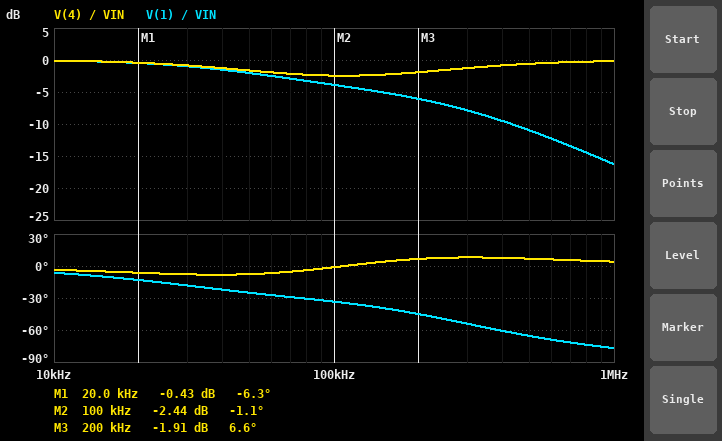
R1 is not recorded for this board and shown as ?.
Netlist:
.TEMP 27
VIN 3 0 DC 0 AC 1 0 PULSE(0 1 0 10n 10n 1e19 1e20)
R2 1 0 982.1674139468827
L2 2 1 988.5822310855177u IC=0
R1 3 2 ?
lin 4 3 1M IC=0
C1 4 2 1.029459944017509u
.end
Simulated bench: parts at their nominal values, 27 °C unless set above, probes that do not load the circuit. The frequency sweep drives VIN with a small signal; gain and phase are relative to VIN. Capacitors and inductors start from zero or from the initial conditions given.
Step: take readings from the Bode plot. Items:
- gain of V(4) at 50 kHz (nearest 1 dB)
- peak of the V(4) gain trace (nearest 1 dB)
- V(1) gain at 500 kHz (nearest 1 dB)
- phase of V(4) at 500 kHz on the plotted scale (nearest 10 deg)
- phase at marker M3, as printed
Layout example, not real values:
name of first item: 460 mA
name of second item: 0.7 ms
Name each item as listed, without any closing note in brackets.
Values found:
gain of V(4) at 50 kHz: -2 dB
peak of the V(4) gain trace: 0 dB
V(1) gain at 500 kHz: -11 dB
phase of V(4) at 500 kHz on the plotted scale: 10 deg
phase at marker M3, as printed: 6.6 deg
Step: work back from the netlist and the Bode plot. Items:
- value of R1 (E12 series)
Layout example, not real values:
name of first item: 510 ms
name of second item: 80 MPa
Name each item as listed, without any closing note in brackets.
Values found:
value of R1: 470 Ω
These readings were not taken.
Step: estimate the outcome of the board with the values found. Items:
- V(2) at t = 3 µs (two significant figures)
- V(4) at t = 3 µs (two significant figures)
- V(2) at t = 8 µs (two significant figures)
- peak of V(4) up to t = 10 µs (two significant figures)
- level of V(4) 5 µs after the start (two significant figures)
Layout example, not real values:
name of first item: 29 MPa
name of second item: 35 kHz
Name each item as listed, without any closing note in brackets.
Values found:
V(2) at t = 3 µs: 850 mV
V(4) at t = 3 µs: 850 mV
V(2) at t = 8 µs: 960 mV
peak of V(4) up to t = 10 µs: 1.0 V
level of V(4) 5 µs after the start: 920 mV
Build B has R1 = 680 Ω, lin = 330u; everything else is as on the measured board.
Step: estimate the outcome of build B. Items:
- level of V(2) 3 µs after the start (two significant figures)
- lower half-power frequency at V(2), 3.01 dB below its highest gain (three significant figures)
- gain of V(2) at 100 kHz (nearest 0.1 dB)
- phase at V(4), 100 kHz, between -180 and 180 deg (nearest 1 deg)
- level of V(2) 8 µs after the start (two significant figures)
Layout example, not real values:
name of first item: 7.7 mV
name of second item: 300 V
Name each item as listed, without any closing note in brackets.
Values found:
level of V(2) 3 µs after the start: 960 mV
lower half-power frequency at V(2), 3.01 dB below its highest gain: 211 Hz
gain of V(2) at 100 kHz: -1.1 dB
phase at V(4), 100 kHz, between -180 and 180 deg: -6 deg
level of V(2) 8 µs after the start: 990 mV
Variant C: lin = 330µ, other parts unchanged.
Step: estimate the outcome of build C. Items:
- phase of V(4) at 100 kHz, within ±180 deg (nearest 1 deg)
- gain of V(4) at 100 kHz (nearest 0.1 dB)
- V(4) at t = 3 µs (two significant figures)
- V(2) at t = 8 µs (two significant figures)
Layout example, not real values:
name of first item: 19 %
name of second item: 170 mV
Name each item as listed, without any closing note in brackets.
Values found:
phase of V(4) at 100 kHz, within ±180 deg: -5 deg
gain of V(4) at 100 kHz: -1.1 dB
V(4) at t = 3 µs: 960 mV
V(2) at t = 8 µs: 990 mV
